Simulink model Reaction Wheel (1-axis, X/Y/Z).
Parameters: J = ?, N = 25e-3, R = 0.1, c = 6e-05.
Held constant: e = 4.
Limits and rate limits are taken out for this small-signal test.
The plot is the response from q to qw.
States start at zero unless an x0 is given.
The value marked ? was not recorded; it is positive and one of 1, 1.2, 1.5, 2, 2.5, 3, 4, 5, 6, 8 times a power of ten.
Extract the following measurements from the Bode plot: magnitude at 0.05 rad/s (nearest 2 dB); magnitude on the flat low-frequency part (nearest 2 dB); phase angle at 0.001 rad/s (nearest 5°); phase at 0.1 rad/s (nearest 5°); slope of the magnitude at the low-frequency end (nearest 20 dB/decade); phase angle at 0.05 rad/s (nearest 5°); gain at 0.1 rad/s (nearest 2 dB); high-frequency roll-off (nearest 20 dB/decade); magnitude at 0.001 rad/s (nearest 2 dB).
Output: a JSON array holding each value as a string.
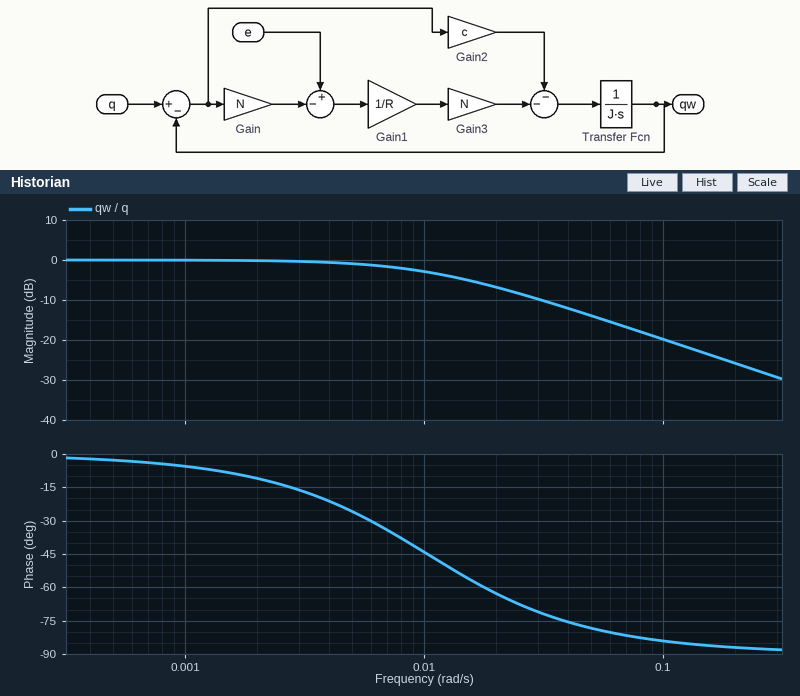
["-14 dB", "0 dB", "-5°", "-85°", "0 dB/decade", "-80°", "-20 dB", "-20 dB/decade", "0 dB"]
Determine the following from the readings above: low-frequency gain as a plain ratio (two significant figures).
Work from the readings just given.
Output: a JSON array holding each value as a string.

["1.0"]
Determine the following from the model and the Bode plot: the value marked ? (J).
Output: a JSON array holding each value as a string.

["0.6"]
